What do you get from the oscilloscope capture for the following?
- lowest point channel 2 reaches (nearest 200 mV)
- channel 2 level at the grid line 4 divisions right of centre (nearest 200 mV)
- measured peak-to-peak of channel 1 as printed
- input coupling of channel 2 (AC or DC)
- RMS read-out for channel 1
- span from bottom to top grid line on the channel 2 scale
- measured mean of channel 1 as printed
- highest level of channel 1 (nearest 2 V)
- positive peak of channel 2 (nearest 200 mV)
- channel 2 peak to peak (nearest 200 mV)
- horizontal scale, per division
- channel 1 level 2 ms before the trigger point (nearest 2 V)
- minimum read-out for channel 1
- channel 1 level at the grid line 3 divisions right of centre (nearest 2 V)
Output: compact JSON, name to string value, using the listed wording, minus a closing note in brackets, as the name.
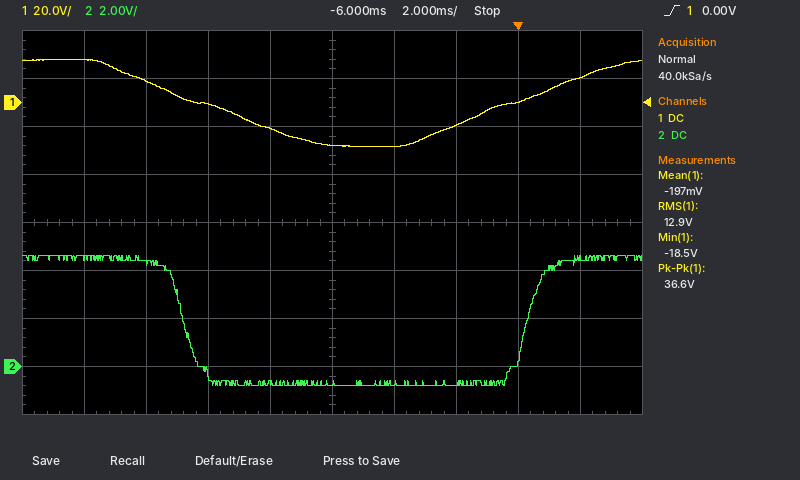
{"lowest point channel 2 reaches": "-800 mV", "channel 2 level at the grid line 4 divisions right of centre": "4.6 V", "measured peak-to-peak of channel 1 as printed": "36.6 V", "input coupling of channel 2": "DC", "RMS read-out for channel 1": "12.9 V", "span from bottom to top grid line on the channel 2 scale": "16 V", "measured mean of channel 1 as printed": "-197 mV", "highest level of channel 1": "18 V", "positive peak of channel 2": "4.6 V", "channel 2 peak to peak": "5.4 V", "horizontal scale, per division": "2 ms", "channel 1 level 2 ms before the trigger point": "-10 V", "minimum read-out for channel 1": "-18.5 V", "channel 1 level at the grid line 3 divisions right of centre": "0 V"}
